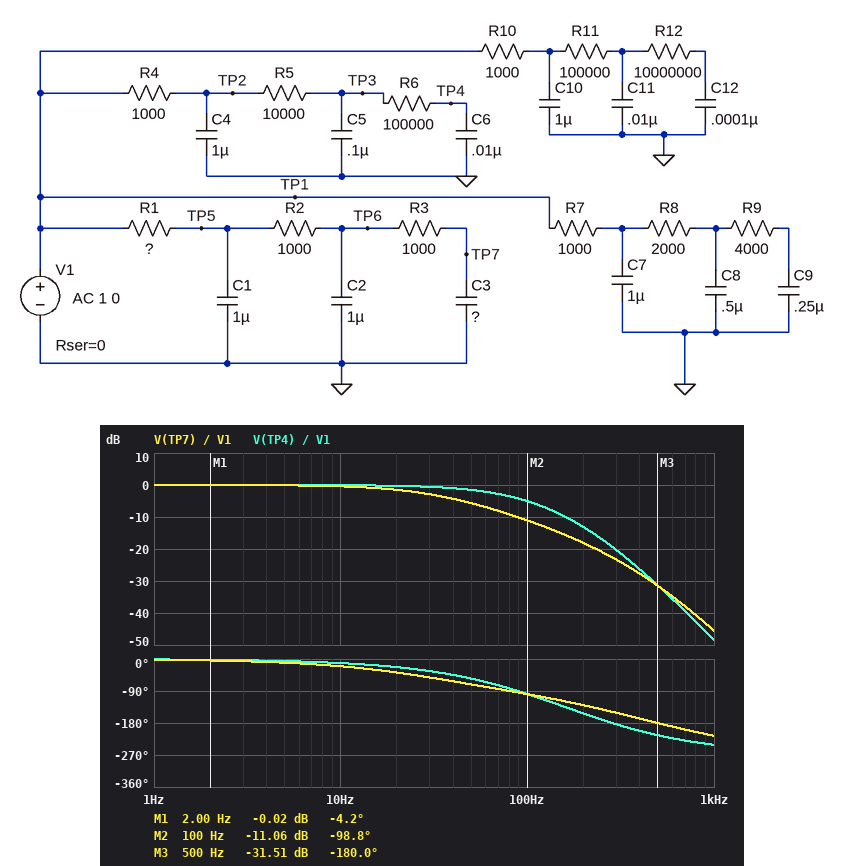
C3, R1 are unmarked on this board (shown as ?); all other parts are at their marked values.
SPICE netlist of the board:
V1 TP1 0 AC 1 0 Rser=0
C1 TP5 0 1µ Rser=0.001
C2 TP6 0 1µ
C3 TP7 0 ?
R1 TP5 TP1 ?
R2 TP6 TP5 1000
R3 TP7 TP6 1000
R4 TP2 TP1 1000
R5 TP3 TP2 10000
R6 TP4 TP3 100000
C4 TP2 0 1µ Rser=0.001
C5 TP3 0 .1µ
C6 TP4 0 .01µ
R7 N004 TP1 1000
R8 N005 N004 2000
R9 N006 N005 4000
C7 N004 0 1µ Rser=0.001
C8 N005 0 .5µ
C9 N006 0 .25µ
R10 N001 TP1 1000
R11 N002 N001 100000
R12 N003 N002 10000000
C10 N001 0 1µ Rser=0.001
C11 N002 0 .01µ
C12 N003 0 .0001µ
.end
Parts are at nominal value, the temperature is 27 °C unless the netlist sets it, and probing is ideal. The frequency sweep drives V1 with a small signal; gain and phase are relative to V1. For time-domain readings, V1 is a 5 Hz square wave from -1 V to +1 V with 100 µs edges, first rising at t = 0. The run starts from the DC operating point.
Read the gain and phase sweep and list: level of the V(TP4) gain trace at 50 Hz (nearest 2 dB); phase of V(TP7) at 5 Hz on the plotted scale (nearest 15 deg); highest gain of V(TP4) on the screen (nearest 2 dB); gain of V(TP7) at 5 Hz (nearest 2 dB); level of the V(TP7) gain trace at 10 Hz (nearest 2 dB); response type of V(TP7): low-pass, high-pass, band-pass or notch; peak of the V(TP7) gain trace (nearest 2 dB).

-2 dB
-15 deg
0 dB
0 dB
0 dB
low-pass
0 dB
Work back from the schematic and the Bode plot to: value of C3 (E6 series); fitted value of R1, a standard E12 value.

330 nF
1.8 kΩ
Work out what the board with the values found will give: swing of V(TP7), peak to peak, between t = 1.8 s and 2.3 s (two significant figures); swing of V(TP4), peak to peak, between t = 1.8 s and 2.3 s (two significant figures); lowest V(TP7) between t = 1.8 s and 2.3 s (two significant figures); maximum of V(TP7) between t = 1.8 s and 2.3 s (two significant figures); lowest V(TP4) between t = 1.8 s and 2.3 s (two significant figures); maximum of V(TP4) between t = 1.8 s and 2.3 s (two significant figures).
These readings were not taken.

2.0 V
2.0 V
-1.0 V
1.0 V
-1.0 V
1.0 V
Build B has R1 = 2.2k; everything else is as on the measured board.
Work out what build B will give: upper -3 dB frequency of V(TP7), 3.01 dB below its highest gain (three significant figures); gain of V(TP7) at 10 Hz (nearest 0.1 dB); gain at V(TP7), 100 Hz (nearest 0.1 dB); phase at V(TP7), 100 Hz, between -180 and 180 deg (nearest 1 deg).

26.2 Hz
-0.6 dB
-12.4 dB
-102 deg
